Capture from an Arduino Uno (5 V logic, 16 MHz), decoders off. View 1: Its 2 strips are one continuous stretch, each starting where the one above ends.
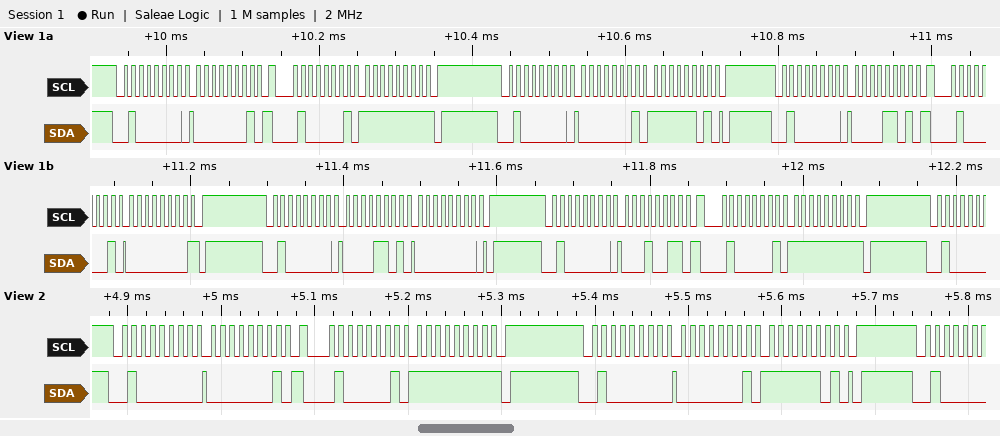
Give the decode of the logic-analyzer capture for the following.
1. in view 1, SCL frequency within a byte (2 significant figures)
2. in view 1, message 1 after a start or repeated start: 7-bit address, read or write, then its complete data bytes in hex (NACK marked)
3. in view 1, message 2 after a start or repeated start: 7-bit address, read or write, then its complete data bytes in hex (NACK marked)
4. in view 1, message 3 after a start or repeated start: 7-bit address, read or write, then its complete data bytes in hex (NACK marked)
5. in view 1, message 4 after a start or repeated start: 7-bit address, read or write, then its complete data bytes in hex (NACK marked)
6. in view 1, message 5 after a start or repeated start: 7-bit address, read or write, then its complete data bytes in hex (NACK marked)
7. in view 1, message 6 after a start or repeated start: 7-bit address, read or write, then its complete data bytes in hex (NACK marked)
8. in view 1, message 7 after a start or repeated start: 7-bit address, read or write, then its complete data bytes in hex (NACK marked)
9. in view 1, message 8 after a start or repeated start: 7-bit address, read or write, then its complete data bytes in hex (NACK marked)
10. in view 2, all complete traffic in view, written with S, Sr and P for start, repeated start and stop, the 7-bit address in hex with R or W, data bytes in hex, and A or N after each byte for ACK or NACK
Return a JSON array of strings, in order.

["100 kHz", "0x20 write: 01", "0x20 read: FF NACK", "0x20 write: 01 FD", "0x20 write: 0D", "0x20 read: 00 NACK", "0x20 write: 0D 00", "0x20 write: 13", "0x20 read: FF NACK", "S 20W A 01 A Sr 20R A FF N P S 20W A 01 A FD A P"]
